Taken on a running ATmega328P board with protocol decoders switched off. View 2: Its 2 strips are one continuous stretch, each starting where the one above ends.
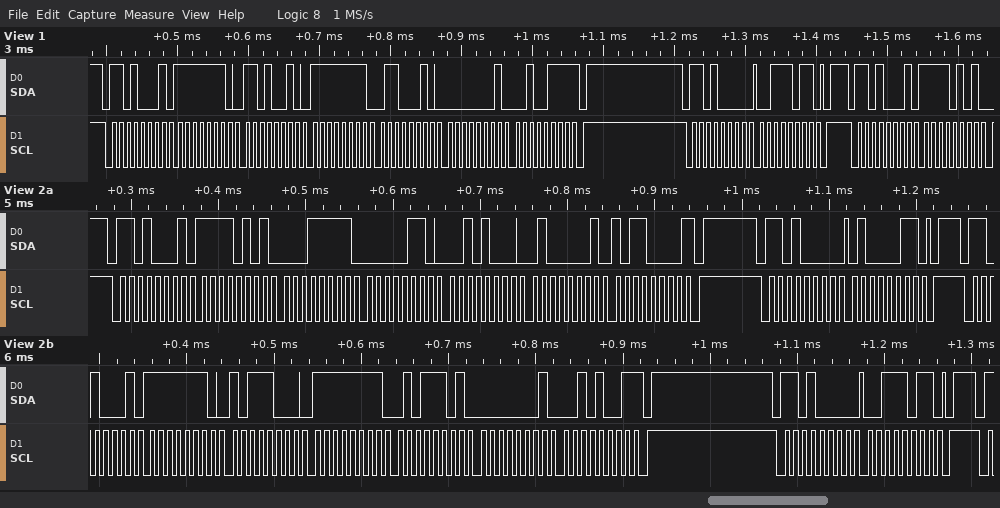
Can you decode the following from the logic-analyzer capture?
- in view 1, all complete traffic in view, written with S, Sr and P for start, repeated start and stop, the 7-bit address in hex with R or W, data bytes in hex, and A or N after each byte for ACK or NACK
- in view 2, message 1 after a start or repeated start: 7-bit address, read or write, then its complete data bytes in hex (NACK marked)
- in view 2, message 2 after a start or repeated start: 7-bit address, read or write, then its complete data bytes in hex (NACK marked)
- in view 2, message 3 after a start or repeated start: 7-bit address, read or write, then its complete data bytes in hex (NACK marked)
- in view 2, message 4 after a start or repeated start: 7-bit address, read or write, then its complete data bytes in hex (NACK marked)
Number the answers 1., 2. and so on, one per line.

1. S 68R A FE A D2 A FF A 62 A 01 A 27 N P S 68W A 3B A P S 68R A F5 A
2. 0x68 read: F5 1F 06 28 41 B0 NACK
3. 0x68 write: 43
4. 0x68 read: FE B8 FF 5D 01 29 NACK
5. 0x68 write: 3B
